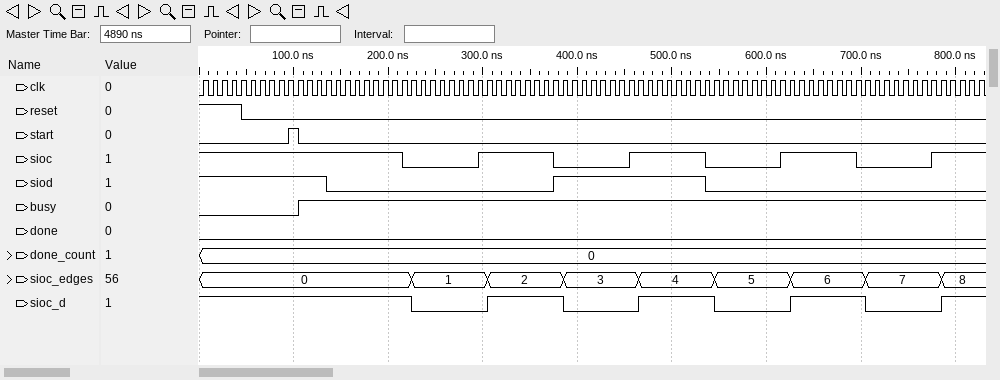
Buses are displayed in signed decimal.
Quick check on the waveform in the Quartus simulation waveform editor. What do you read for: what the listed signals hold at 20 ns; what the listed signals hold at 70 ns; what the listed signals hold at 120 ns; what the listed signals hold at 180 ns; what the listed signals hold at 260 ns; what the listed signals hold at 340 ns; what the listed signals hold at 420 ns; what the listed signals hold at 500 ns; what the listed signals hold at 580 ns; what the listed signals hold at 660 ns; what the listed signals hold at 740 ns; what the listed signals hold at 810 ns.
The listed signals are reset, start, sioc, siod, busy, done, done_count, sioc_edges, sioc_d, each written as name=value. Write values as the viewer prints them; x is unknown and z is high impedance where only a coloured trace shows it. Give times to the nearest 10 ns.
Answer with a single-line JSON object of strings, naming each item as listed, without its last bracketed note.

{"what the listed signals hold at 20 ns": "reset=1, start=0, sioc=1, siod=1, busy=0, done=0, done_count=0, sioc_edges=0, sioc_d=1", "what the listed signals hold at 70 ns": "reset=0, start=0, sioc=1, siod=1, busy=0, done=0, done_count=0, sioc_edges=0, sioc_d=1", "what the listed signals hold at 120 ns": "reset=0, start=0, sioc=1, siod=1, busy=1, done=0, done_count=0, sioc_edges=0, sioc_d=1", "what the listed signals hold at 180 ns": "reset=0, start=0, sioc=1, siod=0, busy=1, done=0, done_count=0, sioc_edges=0, sioc_d=1", "what the listed signals hold at 260 ns": "reset=0, start=0, sioc=0, siod=0, busy=1, done=0, done_count=0, sioc_edges=1, sioc_d=0", "what the listed signals hold at 340 ns": "reset=0, start=0, sioc=1, siod=0, busy=1, done=0, done_count=0, sioc_edges=2, sioc_d=1", "what the listed signals hold at 420 ns": "reset=0, start=0, sioc=0, siod=1, busy=1, done=0, done_count=0, sioc_edges=3, sioc_d=0", "what the listed signals hold at 500 ns": "reset=0, start=0, sioc=1, siod=1, busy=1, done=0, done_count=0, sioc_edges=4, sioc_d=1", "what the listed signals hold at 580 ns": "reset=0, start=0, sioc=0, siod=0, busy=1, done=0, done_count=0, sioc_edges=5, sioc_d=0", "what the listed signals hold at 660 ns": "reset=0, start=0, sioc=1, siod=0, busy=1, done=0, done_count=0, sioc_edges=6, sioc_d=1", "what the listed signals hold at 740 ns": "reset=0, start=0, sioc=0, siod=0, busy=1, done=0, done_count=0, sioc_edges=7, sioc_d=0", "what the listed signals hold at 810 ns": "reset=0, start=0, sioc=1, siod=0, busy=1, done=0, done_count=0, sioc_edges=8, sioc_d=1"}
